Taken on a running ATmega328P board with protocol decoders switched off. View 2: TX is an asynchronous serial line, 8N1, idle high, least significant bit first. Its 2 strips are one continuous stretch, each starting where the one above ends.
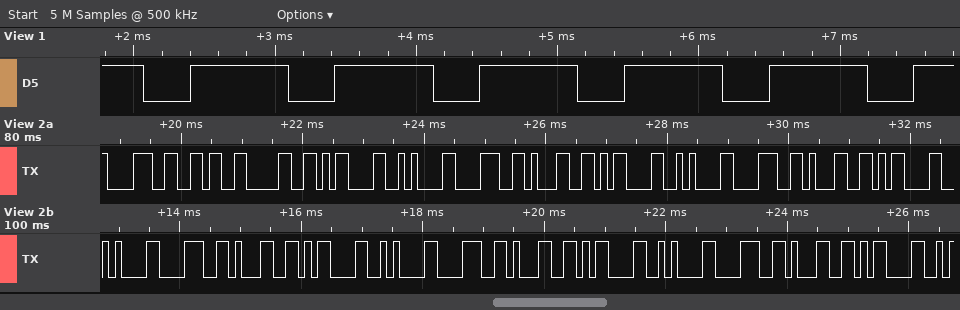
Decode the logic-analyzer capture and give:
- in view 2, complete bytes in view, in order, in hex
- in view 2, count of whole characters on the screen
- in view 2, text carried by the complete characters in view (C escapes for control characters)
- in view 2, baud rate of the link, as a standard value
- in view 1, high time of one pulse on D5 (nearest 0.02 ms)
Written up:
38 36 30 0D 0A 38 31 0D 0A 38 31 0D 0A 38 31 0D 0A 38 31 0D 0A 38 31 0D
24
"860\r\n81\r\n81\r\n81\r\n81\r\n81\r"
9600 baud
0.70 ms
